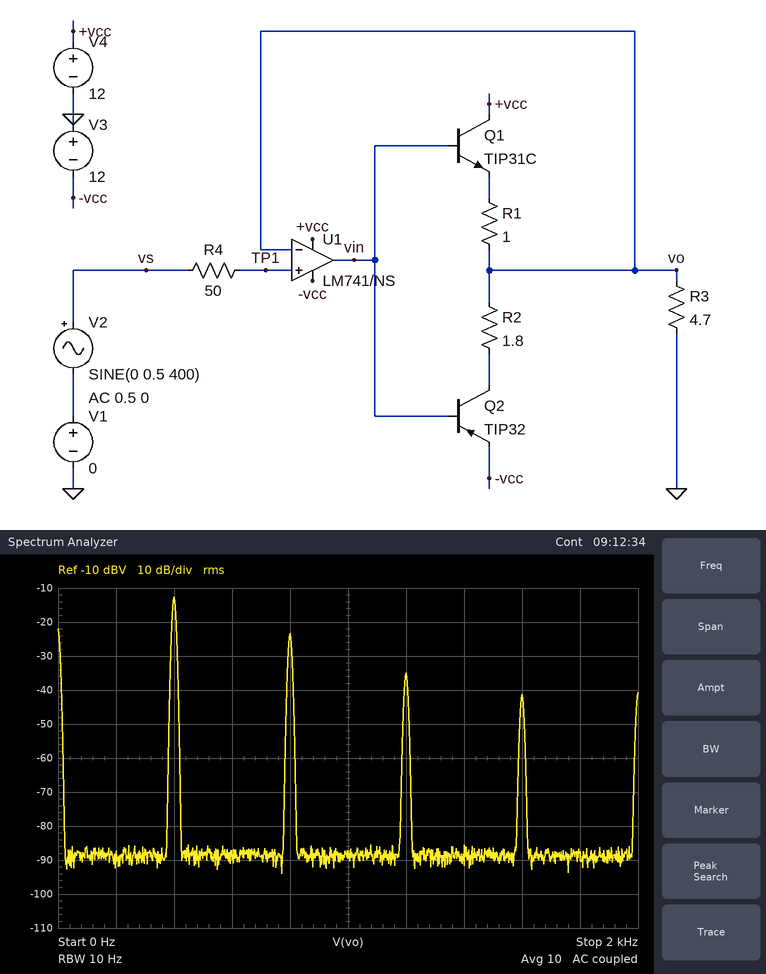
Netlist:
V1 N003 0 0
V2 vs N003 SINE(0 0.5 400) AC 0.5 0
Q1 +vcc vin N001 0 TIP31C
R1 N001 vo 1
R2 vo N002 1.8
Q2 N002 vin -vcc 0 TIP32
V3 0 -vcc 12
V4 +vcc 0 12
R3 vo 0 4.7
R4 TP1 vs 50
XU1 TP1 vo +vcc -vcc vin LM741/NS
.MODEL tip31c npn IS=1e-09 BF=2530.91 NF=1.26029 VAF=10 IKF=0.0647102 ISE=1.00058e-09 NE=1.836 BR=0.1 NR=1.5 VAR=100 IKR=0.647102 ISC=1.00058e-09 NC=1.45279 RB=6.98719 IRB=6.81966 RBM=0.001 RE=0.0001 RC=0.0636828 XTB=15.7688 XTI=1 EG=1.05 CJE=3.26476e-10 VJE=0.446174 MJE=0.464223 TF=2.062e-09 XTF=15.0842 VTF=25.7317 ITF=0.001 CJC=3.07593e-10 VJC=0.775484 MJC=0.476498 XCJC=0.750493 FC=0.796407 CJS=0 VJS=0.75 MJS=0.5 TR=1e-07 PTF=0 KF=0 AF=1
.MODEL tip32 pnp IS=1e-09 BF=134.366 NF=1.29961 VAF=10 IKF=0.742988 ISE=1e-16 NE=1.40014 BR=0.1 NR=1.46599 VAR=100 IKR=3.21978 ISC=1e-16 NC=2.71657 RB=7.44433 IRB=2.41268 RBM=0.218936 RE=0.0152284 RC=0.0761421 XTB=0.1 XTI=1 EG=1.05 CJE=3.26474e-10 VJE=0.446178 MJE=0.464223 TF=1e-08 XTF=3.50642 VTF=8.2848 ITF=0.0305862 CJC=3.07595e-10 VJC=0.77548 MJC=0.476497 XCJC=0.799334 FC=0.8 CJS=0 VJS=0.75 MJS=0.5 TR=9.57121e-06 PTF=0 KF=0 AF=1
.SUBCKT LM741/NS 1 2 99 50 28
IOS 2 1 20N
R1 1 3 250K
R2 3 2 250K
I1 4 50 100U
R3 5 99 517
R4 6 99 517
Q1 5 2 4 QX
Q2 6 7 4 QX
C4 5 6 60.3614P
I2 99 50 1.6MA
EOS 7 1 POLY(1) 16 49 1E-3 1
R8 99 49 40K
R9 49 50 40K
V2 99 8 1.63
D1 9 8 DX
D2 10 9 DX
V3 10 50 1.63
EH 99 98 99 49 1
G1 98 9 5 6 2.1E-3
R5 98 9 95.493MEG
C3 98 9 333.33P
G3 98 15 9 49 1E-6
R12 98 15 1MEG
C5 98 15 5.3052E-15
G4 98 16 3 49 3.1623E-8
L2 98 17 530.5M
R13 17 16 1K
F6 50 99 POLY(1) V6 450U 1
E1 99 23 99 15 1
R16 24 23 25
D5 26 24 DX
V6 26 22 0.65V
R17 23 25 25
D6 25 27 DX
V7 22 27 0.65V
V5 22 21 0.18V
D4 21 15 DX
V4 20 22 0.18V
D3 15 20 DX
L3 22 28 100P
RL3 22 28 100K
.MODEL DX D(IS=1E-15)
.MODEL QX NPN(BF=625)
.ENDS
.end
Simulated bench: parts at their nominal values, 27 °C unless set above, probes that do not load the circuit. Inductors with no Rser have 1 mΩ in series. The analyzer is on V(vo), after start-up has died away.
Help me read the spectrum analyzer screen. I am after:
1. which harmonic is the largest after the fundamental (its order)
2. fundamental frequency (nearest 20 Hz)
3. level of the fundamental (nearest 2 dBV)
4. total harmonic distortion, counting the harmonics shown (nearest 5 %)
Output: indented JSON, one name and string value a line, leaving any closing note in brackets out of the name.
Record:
{
  "which harmonic is the largest after the fundamental": "2",
  "fundamental frequency": "400 Hz",
  "level of the fundamental": "-12 dBV",
  "total harmonic distortion, counting the harmonics shown": "30 %"
}
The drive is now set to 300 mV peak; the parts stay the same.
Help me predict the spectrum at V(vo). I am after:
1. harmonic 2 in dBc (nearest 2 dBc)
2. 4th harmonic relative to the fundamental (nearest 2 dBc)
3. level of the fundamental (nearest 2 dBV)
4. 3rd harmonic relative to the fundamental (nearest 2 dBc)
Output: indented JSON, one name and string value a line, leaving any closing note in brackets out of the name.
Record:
{
  "harmonic 2 in dBc": "-14 dBc",
  "4th harmonic relative to the fundamental": "-42 dBc",
  "level of the fundamental": "-16 dBV",
  "3rd harmonic relative to the fundamental": "-20 dBc"
}
